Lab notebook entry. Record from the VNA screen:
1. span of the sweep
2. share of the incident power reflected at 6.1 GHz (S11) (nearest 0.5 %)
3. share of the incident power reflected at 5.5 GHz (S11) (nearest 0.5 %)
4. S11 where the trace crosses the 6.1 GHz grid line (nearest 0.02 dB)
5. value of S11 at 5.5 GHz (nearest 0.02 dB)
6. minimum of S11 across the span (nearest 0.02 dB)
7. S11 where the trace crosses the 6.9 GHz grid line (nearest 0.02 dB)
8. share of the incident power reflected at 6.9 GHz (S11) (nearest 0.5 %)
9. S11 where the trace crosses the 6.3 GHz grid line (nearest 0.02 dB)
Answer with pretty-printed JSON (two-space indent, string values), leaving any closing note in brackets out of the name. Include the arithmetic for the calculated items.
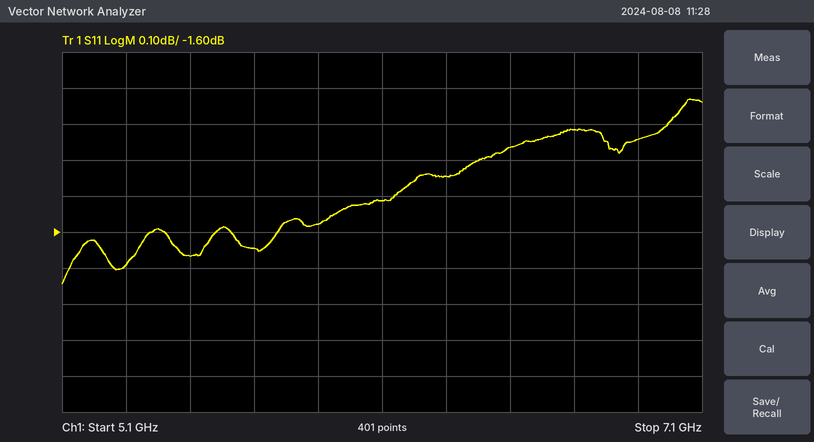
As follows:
{
  "span of the sweep": "2 GHz",
  "share of the incident power reflected at 6.1 GHz (S11)": "10^(-1.52/10) ≈ 70.5 %",
  "share of the incident power reflected at 5.5 GHz (S11)": "10^(-1.66/10) ≈ 68.2 %, so 68.0 % to the nearest 0.5 %",
  "S11 where the trace crosses the 6.1 GHz grid line": "-1.52 dB",
  "value of S11 at 5.5 GHz": "-1.66 dB",
  "minimum of S11 across the span": "-1.74 dB",
  "S11 where the trace crosses the 6.9 GHz grid line": "-1.34 dB",
  "share of the incident power reflected at 6.9 GHz (S11)": "10^(-1.34/10) ≈ 73.5 %",
  "S11 where the trace crosses the 6.3 GHz grid line": "-1.44 dB"
}
